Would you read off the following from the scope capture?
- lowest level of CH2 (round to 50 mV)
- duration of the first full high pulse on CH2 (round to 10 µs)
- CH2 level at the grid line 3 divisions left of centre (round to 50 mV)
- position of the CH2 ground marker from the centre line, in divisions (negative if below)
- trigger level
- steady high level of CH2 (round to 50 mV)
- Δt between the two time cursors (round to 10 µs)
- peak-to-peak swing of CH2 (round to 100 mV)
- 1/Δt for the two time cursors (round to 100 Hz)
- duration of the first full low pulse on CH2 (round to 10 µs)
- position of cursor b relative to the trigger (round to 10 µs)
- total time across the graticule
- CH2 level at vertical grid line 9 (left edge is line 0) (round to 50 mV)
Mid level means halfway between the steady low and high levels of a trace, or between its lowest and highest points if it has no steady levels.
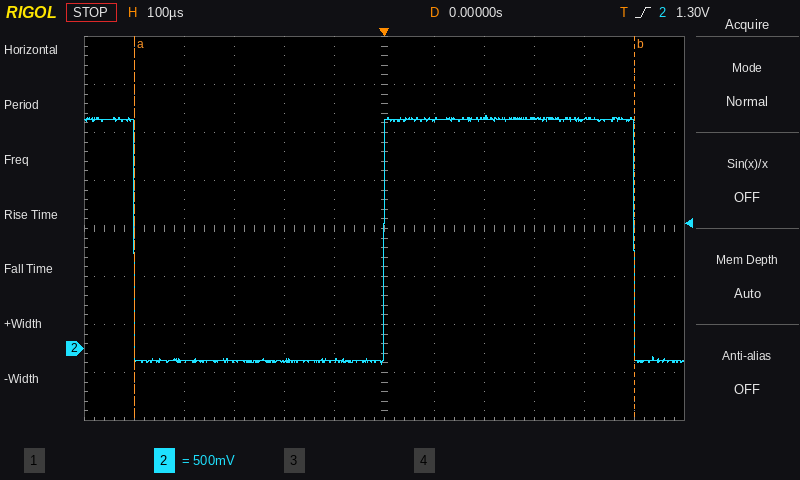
-150 mV
500 µs
-150 mV
-2.5 div
1.30 V
2.40 V
1.00 ms
2.60 V
1.0 kHz
500 µs
+500 µs
1.2 ms
2.40 V
